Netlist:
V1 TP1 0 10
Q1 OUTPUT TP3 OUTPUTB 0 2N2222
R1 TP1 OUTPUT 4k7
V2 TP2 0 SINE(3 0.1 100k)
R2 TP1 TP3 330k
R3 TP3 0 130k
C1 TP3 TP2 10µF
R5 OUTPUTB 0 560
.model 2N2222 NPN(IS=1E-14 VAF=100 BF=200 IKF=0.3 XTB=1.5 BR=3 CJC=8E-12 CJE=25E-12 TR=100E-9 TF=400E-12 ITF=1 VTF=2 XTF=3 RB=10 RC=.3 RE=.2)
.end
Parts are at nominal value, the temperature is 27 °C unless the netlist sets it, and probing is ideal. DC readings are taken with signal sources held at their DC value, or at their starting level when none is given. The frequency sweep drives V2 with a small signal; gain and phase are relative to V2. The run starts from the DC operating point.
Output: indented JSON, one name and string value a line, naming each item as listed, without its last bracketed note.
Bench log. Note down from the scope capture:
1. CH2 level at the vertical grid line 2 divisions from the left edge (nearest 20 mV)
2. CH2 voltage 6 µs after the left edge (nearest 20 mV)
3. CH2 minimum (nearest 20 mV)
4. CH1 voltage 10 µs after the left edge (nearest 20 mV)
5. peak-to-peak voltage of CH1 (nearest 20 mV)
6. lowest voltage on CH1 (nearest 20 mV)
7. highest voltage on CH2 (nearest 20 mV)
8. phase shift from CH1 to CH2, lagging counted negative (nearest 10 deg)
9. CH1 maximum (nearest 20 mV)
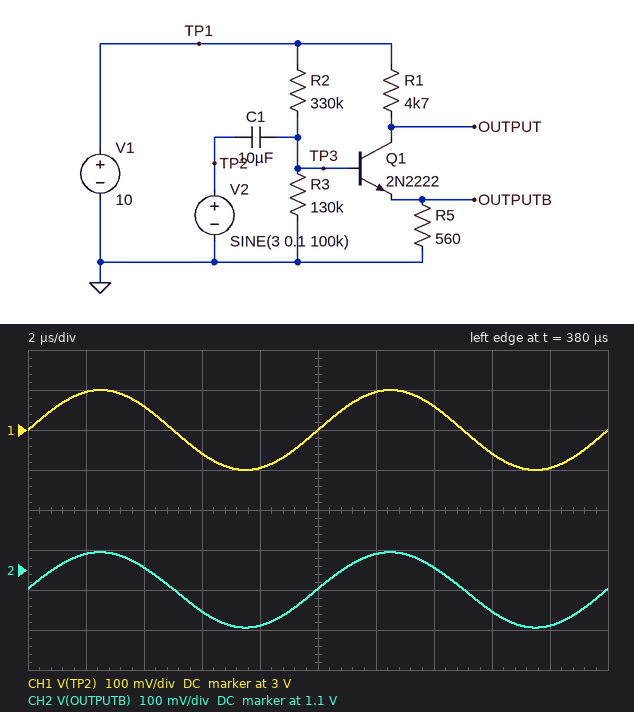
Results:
{
  "CH2 level at the vertical grid line 2 divisions from the left edge": "1.10 V",
  "CH2 voltage 6 µs after the left edge": "1.00 V",
  "CH2 minimum": "960 mV",
  "CH1 voltage 10 µs after the left edge": "3.00 V",
  "peak-to-peak voltage of CH1": "200 mV",
  "lowest voltage on CH1": "2.90 V",
  "highest voltage on CH2": "1.14 V",
  "phase shift from CH1 to CH2, lagging counted negative": "0 deg",
  "CH1 maximum": "3.10 V"
}
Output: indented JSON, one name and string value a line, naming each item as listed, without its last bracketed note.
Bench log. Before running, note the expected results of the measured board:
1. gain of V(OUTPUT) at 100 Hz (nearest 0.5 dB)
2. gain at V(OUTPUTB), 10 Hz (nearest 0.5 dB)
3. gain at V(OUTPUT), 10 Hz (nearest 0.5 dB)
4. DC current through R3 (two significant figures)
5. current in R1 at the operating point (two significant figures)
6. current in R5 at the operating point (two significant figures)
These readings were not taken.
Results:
{
  "gain of V(OUTPUT) at 100 Hz": "14.5 dB",
  "gain at V(OUTPUTB), 10 Hz": "-3.0 dB",
  "gain at V(OUTPUT), 10 Hz": "12.0 dB",
  "DC current through R3": "13 µA",
  "current in R1 at the operating point": "1.9 mA",
  "current in R5 at the operating point": "1.9 mA"
}
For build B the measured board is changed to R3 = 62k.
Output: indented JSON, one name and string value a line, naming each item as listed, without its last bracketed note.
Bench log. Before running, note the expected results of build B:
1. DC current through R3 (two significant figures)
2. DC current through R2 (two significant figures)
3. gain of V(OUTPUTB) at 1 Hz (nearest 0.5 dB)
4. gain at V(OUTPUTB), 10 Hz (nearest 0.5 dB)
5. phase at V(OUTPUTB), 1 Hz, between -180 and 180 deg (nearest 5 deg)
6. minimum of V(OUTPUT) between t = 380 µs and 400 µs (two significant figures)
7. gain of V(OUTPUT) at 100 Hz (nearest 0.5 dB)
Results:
{
  "DC current through R3": "21 µA",
  "DC current through R2": "26 µA",
  "gain of V(OUTPUTB) at 1 Hz": "-1.0 dB",
  "gain at V(OUTPUTB), 10 Hz": "-0.5 dB",
  "phase at V(OUTPUTB), 1 Hz, between -180 and 180 deg": "25 deg",
  "minimum of V(OUTPUT) between t = 380 µs and 400 µs": "3.9 V",
  "gain of V(OUTPUT) at 100 Hz": "18.0 dB"
}
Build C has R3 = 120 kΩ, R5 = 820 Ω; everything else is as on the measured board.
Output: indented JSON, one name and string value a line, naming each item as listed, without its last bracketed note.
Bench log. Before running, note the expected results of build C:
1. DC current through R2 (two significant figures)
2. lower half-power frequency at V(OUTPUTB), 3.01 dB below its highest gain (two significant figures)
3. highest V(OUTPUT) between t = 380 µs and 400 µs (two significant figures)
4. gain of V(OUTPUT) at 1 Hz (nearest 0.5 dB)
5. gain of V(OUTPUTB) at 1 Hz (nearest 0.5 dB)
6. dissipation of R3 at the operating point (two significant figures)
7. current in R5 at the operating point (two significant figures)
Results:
{
  "DC current through R2": "24 µA",
  "lower half-power frequency at V(OUTPUTB), 3.01 dB below its highest gain": "280 mHz",
  "highest V(OUTPUT) between t = 380 µs and 400 µs": "3.1 V",
  "gain of V(OUTPUT) at 1 Hz": "14.5 dB",
  "gain of V(OUTPUTB) at 1 Hz": "-0.5 dB",
  "dissipation of R3 at the operating point": "32 µW",
  "current in R5 at the operating point": "1.6 mA"
}
